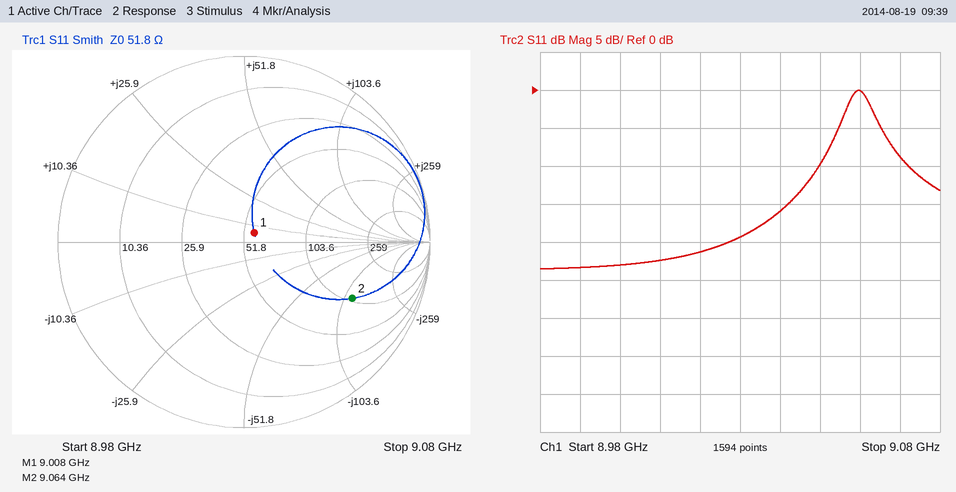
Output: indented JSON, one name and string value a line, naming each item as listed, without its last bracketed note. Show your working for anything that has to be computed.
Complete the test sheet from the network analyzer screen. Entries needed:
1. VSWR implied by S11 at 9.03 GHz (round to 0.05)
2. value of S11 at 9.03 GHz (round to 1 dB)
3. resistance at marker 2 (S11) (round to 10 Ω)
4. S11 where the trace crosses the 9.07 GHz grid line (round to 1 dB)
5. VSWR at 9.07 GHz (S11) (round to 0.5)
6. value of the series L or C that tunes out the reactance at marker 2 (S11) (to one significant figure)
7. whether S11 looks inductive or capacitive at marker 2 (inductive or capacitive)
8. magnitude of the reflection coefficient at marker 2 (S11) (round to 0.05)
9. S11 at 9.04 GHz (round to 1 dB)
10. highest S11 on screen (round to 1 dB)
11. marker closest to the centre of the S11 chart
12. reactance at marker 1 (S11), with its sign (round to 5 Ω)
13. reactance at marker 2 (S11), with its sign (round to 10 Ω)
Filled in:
{
  "VSWR implied by S11 at 9.03 GHz": "|Γ| = 10^(-19/20) = 0.1122; VSWR = (1 + 0.1122)/(1 − 0.1122) ≈ 1.25",
  "value of S11 at 9.03 GHz": "-19 dB",
  "resistance at marker 2 (S11)": "110 Ω",
  "S11 where the trace crosses the 9.07 GHz grid line": "-9 dB",
  "VSWR at 9.07 GHz (S11)": "|Γ| = 10^(-9/20) = 0.3548; VSWR = (1 + 0.3548)/(1 − 0.3548) ≈ 2.10, so 2.0 to the nearest 0.5",
  "value of the series L or C that tunes out the reactance at marker 2 (S11)": "L = 120 Ω/(2π × 9.064 GHz) ≈ 2 nH",
  "whether S11 looks inductive or capacitive at marker 2": "capacitive",
  "magnitude of the reflection coefficient at marker 2 (S11)": "0.65",
  "S11 at 9.04 GHz": "-16 dB",
  "highest S11 on screen": "0 dB",
  "marker closest to the centre of the S11 chart": "marker 1",
  "reactance at marker 1 (S11), with its sign": "+5 Ω",
  "reactance at marker 2 (S11), with its sign": "-120 Ω"
}
